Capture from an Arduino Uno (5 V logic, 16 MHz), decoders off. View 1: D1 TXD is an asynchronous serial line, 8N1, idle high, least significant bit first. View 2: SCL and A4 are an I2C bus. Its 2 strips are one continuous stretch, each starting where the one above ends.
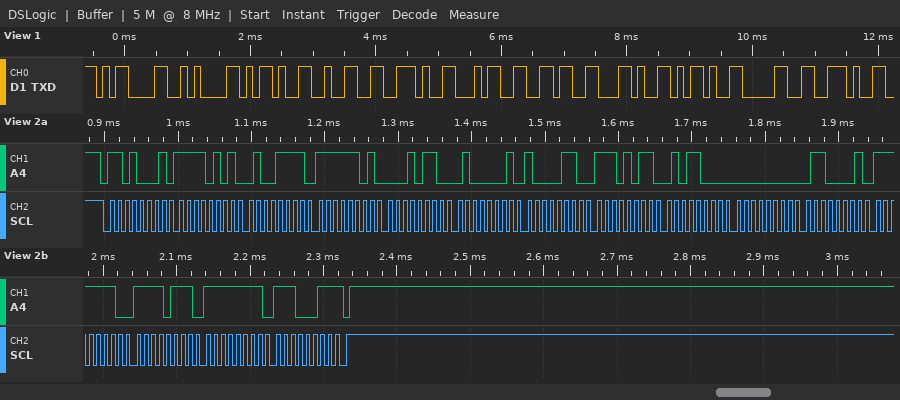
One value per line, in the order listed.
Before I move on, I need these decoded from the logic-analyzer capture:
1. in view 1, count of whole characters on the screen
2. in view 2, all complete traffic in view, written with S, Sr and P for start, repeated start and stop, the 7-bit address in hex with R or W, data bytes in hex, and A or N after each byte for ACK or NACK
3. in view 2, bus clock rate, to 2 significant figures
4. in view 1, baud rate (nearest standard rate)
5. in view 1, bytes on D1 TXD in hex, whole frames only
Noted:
11
S 68R A F5 A 4F A FD A 16 A 41 A 86 A EB A 58 A 00 A 61 A FE A F7 A FF A E3 N P
100 kHz
9600 baud
0D 0A 2D 32 2E 34 36 2C 2D 30 2E
